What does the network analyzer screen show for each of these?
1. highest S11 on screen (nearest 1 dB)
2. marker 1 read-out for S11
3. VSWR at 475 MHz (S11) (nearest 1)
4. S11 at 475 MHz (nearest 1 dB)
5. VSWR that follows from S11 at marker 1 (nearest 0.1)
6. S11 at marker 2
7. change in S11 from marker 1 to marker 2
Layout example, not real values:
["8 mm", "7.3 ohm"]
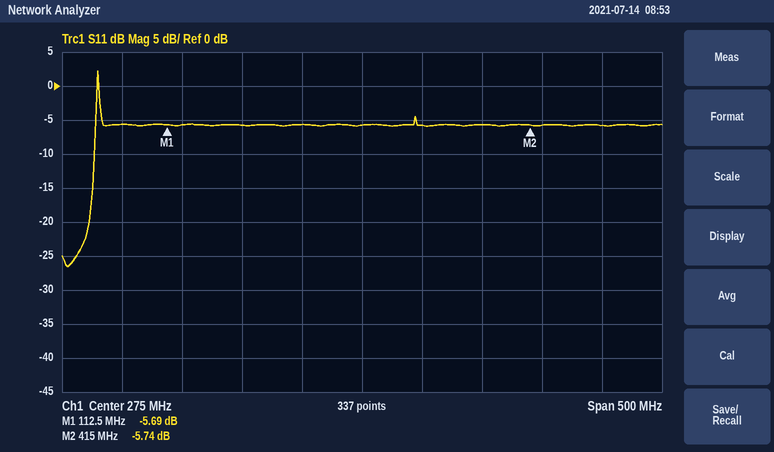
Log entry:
["2 dB", "-5.69 dB", "3", "-6 dB", "3.2", "-5.74 dB", "-0.05 dB"]
